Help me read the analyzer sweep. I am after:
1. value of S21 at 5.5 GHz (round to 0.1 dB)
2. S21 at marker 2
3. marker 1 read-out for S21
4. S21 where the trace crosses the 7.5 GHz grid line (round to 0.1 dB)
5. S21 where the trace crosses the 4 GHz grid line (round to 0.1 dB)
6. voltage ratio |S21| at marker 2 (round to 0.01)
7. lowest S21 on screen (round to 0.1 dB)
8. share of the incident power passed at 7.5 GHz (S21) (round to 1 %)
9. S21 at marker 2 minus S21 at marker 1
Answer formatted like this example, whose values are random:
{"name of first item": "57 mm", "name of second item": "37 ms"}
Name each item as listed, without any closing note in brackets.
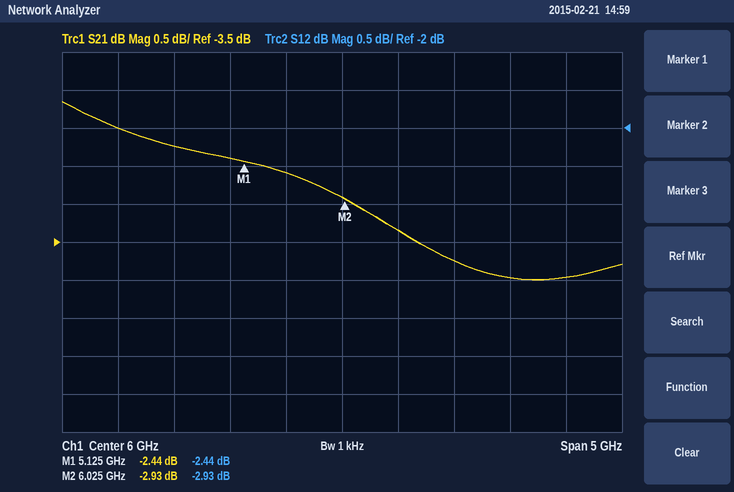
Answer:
{"value of S21 at 5.5 GHz": "-2.6 dB", "S21 at marker 2": "-2.93 dB", "marker 1 read-out for S21": "-2.44 dB", "S21 where the trace crosses the 7.5 GHz grid line": "-4.0 dB", "S21 where the trace crosses the 4 GHz grid line": "-2.0 dB", "voltage ratio |S21| at marker 2": "0.71", "lowest S21 on screen": "-4.0 dB", "share of the incident power passed at 7.5 GHz (S21)": "40 %", "S21 at marker 2 minus S21 at marker 1": "-0.49 dB"}
